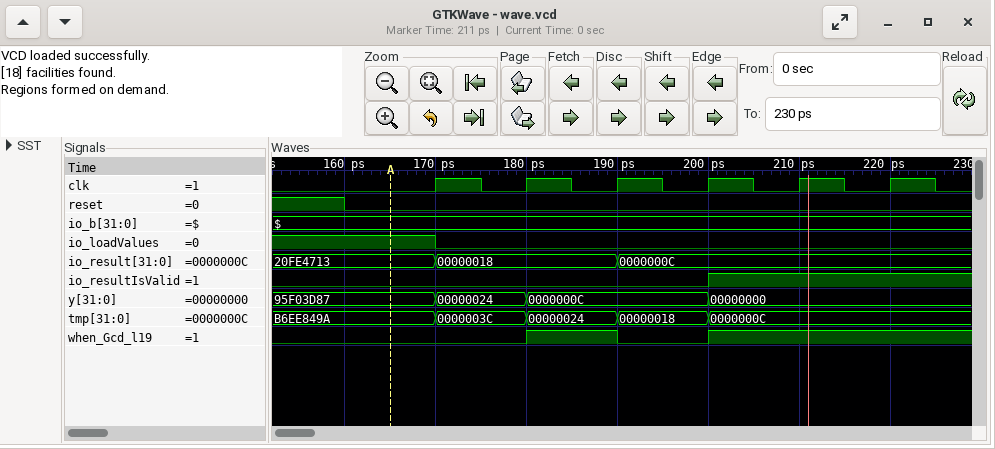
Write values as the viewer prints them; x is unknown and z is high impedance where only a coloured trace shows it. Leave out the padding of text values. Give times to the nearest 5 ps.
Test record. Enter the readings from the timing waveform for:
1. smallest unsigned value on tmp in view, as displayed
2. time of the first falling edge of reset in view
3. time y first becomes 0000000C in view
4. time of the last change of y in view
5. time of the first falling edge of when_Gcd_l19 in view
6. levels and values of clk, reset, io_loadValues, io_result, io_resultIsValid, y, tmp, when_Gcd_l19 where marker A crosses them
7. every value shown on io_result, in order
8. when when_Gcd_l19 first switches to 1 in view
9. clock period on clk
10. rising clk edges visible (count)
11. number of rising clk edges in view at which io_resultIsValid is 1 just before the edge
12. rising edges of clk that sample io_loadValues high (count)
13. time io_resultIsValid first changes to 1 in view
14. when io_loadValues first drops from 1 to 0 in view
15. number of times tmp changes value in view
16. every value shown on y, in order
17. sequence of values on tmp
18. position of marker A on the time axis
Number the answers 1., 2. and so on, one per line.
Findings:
1. 0000000C
2. 160 ps
3. 180 ps
4. 200 ps
5. 190 ps
6. clk=0, reset=0, io_loadValues=1, io_result=20FE4713, io_resultIsValid=0, y=95F03D87, tmp=B6EE849A, when_Gcd_l19=0
7. 20FE4713, 00000018, 0000000C
8. 180 ps
9. 10 ps
10. 6
11. 2
12. 1
13. 200 ps
14. 170 ps
15. 4
16. 95F03D87, 00000024, 0000000C, 00000000
17. B6EE849A, 0000003C, 00000024, 00000018, 0000000C
18. 165 ps
